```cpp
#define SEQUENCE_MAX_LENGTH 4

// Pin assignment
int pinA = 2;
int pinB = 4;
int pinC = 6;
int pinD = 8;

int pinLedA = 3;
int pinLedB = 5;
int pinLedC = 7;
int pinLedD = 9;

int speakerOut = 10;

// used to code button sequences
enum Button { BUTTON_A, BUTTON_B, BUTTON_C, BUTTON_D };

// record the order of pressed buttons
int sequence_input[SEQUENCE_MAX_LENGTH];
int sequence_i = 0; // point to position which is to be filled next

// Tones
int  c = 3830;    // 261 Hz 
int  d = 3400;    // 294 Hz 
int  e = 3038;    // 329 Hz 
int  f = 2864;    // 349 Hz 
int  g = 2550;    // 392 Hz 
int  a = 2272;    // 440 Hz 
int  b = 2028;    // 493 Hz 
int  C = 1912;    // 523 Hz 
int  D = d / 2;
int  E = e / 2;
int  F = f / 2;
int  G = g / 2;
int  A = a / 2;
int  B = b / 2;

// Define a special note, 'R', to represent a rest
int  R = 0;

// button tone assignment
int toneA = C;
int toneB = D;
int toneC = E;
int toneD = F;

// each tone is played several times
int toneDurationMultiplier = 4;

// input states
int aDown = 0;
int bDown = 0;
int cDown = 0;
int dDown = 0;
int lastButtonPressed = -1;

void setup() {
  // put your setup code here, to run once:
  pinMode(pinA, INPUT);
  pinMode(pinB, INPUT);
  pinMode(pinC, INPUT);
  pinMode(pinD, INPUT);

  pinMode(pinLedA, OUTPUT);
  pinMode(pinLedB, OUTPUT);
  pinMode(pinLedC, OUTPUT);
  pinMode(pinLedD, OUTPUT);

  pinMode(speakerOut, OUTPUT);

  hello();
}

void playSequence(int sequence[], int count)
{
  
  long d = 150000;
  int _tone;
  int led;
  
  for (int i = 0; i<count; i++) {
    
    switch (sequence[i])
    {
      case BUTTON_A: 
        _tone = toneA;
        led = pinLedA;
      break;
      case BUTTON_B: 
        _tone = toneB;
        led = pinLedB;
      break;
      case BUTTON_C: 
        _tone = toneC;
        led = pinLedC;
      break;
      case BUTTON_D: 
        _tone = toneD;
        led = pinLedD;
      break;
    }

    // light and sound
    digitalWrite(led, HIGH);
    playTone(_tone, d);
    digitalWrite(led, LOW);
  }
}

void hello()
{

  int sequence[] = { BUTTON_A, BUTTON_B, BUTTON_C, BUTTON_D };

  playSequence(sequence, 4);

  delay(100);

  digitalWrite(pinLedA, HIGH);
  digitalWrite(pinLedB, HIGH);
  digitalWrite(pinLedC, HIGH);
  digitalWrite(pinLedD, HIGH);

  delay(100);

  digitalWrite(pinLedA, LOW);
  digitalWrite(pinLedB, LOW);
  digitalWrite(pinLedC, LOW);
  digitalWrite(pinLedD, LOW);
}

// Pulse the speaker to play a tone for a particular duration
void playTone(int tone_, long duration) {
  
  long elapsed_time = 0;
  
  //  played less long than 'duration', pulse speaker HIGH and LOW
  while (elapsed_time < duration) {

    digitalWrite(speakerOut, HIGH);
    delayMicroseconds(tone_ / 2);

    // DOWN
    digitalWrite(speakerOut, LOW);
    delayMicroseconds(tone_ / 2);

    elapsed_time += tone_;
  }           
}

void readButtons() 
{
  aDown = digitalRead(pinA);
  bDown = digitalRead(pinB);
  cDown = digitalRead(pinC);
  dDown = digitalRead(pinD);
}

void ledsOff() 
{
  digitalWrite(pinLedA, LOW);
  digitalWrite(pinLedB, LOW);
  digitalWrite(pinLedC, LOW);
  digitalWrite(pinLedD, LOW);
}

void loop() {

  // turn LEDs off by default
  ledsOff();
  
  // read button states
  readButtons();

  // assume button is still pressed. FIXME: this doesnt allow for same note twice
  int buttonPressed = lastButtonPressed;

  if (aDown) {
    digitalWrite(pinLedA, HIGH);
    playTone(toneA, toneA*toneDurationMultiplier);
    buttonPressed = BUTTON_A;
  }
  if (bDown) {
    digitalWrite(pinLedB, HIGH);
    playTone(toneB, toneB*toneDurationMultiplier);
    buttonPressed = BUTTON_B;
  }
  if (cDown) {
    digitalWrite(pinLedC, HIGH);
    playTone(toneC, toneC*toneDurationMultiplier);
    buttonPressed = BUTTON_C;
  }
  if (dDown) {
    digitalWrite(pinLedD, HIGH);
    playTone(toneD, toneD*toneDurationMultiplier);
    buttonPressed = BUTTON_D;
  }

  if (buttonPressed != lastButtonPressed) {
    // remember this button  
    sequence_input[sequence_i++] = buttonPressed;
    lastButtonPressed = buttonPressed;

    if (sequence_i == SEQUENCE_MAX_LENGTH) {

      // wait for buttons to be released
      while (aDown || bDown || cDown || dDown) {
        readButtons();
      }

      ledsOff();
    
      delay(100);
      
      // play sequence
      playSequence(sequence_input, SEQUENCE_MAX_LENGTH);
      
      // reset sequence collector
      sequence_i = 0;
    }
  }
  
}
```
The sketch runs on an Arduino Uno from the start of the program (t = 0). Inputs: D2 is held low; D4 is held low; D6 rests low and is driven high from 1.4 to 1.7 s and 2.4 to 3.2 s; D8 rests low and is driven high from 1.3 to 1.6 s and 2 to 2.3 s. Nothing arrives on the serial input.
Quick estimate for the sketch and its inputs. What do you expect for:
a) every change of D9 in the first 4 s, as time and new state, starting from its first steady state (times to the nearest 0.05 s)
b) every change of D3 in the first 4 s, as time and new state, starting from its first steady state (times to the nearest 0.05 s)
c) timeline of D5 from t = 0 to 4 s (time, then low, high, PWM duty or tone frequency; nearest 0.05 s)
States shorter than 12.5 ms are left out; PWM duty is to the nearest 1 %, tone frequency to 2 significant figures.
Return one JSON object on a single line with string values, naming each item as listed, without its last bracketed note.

{"every change of D9 in the first 4 s, as time and new state, starting from its first steady state": "0 s low; 0.45 s high; 0.6 s low; 0.7 s high; 0.8 s low; 1.3 s tone 110 Hz; 1.6 s low; 2 s tone 170 Hz; 2.3 s low; 3.3 s high; 3.45 s low; 3.6 s high; 3.75 s low", "every change of D3 in the first 4 s, as time and new state, starting from its first steady state": "0 s high; 0.15 s low; 0.7 s high; 0.8 s low", "timeline of D5 from t = 0 to 4 s": "0 s low; 0.15 s high; 0.3 s low; 0.7 s high; 0.8 s low"}
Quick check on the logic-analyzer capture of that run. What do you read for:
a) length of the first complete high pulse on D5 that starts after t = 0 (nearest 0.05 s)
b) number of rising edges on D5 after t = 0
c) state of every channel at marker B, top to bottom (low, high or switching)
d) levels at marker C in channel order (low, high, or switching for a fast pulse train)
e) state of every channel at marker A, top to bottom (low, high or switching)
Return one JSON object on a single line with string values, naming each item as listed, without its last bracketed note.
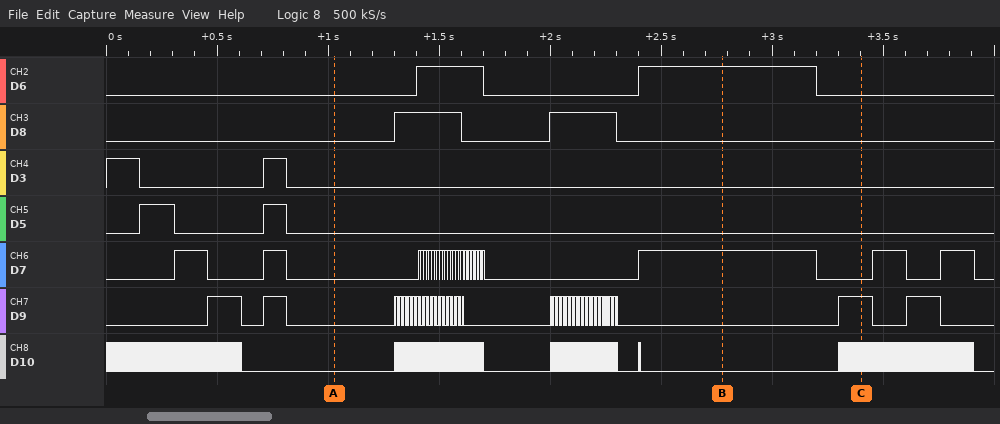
{"length of the first complete high pulse on D5 that starts after t = 0": "0.15 s", "number of rising edges on D5 after t = 0": "2", "state of every channel at marker B, top to bottom": "D6 high, D8 low, D3 low, D5 low, D7 high, D9 low, D10 low", "levels at marker C in channel order": "D6 low, D8 low, D3 low, D5 low, D7 low, D9 high, D10 switching", "state of every channel at marker A, top to bottom": "D6 low, D8 low, D3 low, D5 low, D7 low, D9 low, D10 low"}
